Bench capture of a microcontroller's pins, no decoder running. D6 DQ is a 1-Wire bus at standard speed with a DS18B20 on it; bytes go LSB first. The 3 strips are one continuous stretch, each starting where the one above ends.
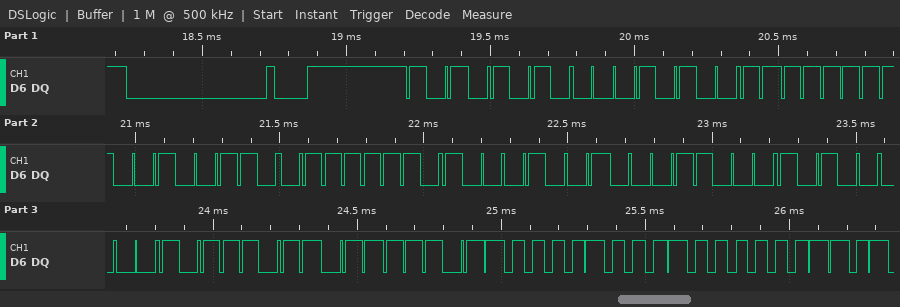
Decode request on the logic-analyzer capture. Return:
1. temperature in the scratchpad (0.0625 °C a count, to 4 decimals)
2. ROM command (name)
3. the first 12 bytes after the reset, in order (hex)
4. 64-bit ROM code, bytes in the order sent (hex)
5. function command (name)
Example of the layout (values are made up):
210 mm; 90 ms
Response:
34.0625 °C; Match ROM; 55 28 FF 64 7E 91 18 05 DD BE 21 02; 28 FF 64 7E 91 18 05 DD; Read Scratchpad
